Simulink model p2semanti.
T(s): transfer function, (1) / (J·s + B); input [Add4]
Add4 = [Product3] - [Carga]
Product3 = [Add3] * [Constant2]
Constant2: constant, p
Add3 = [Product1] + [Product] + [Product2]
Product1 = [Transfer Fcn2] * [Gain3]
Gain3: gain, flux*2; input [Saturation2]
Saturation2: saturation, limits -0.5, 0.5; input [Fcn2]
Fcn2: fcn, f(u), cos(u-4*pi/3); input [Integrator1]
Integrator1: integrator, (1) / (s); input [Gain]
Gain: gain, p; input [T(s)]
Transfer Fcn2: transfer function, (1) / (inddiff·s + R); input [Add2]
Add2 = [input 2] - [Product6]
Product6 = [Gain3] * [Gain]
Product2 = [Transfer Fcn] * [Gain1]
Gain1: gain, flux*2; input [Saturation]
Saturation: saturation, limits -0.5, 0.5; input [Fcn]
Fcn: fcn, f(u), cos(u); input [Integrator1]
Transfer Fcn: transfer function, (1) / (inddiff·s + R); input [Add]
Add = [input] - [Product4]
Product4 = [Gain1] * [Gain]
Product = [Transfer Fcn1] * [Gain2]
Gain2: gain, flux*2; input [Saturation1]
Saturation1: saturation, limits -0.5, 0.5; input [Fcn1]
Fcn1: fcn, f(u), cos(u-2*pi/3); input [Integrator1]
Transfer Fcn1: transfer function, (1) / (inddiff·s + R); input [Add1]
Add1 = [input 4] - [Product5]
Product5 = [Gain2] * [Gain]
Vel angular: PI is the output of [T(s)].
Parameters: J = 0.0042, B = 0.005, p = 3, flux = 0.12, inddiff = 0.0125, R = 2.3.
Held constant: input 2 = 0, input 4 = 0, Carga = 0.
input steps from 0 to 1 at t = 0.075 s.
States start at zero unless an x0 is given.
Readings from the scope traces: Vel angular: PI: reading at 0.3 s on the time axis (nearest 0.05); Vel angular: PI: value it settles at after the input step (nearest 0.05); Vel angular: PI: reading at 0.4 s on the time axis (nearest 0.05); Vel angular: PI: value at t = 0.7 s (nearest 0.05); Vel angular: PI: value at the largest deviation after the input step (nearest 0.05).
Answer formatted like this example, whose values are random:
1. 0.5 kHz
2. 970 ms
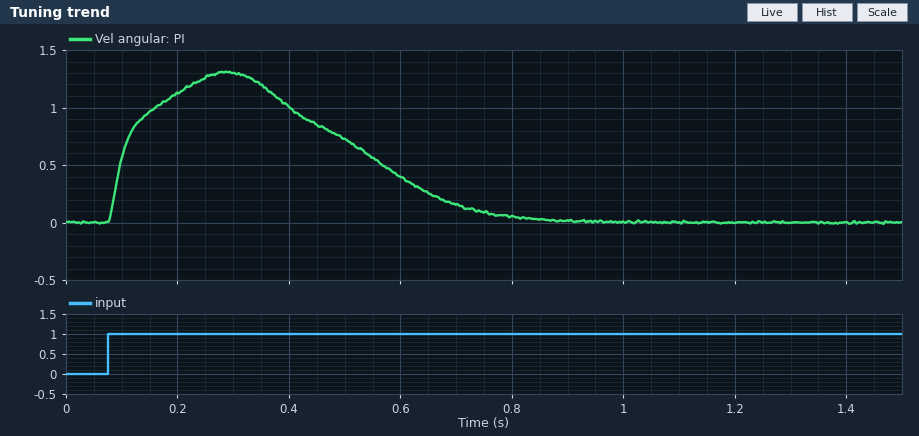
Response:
1. 1.30
2. 0.00
3. 1.00
4. 0.15
5. 1.30
